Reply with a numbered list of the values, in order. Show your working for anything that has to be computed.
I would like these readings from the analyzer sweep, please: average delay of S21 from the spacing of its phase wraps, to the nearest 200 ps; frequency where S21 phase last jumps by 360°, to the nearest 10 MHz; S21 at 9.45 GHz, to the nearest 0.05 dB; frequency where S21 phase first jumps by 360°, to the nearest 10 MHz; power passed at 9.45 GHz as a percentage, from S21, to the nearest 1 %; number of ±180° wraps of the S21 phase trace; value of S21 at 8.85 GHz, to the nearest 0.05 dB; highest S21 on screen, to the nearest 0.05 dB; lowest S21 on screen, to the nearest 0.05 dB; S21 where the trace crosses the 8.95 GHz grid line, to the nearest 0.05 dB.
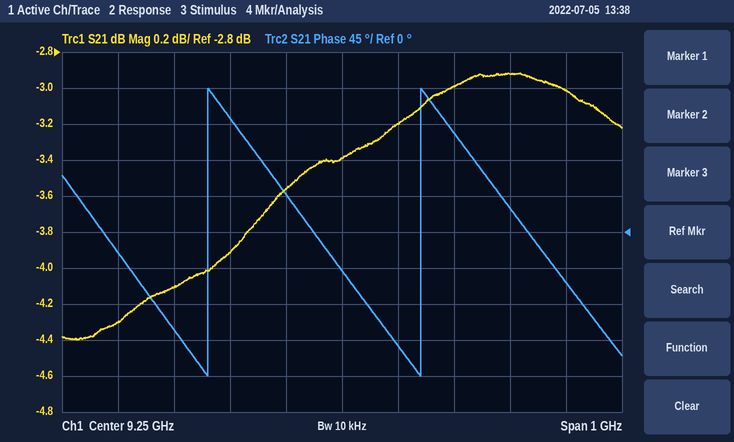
1. 1 cycle / (9.39 GHz − 9.01 GHz) ≈ 2.6 ns
2. 9.39 GHz
3. -3.00 dB
4. 9.01 GHz
5. 10^(-3/10) ≈ 50 %
6. 2
7. -4.30 dB
8. -2.90 dB
9. -4.40 dB
10. -4.10 dB
